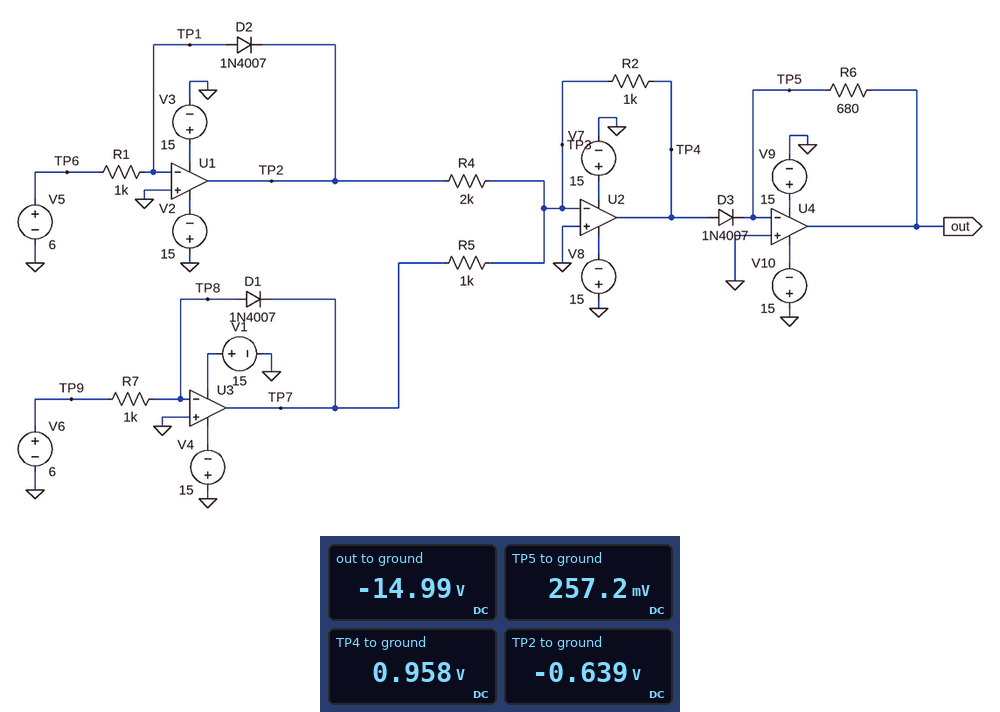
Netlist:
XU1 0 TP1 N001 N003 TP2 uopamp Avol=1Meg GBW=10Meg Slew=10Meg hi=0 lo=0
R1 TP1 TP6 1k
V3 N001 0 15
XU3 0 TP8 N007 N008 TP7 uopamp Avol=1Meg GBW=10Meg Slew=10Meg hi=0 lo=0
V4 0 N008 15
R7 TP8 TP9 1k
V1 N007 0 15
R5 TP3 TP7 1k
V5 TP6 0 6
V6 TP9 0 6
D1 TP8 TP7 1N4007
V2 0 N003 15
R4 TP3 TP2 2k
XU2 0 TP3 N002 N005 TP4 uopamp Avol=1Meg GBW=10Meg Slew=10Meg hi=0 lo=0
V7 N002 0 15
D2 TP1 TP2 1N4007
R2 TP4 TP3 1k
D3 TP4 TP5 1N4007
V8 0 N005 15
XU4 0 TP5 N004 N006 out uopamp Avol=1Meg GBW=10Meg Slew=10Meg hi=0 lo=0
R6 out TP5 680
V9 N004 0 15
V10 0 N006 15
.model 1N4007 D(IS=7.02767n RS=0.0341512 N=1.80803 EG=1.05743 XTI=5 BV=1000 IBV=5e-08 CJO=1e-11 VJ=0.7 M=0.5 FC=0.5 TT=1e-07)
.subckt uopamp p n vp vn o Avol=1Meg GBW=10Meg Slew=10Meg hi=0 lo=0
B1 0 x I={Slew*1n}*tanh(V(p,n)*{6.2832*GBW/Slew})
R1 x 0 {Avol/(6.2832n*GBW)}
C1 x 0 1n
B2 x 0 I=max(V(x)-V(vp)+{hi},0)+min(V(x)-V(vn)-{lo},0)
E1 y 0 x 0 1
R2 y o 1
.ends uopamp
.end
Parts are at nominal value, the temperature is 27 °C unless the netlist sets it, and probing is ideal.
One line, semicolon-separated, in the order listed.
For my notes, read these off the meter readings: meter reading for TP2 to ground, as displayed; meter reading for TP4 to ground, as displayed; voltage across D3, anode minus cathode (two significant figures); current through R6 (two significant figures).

-0.639 V; 0.958 V; 700 mV; 22 mA
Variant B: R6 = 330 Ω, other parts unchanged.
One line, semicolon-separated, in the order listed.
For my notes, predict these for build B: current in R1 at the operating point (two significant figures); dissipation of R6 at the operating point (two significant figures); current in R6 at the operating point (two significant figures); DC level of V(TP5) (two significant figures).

6.0 mA; 700 mW; 46 mA; 220 mV
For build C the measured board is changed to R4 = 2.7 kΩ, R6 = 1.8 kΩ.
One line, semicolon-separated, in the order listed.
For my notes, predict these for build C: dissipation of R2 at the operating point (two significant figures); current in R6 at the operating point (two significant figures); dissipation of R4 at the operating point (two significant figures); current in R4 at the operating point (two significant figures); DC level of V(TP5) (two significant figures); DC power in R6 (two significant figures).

770 µW; 8.5 mA; 150 µW; 240 µA; 220 mV; 130 mW
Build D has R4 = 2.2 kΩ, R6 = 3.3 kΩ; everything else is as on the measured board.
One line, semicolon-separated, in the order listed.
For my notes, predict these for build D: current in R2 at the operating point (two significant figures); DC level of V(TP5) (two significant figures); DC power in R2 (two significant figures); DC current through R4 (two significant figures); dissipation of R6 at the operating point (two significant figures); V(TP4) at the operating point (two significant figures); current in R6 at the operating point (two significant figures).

930 µA; 300 mV; 860 µW; 290 µA; 71 mW; 930 mV; 4.6 mA
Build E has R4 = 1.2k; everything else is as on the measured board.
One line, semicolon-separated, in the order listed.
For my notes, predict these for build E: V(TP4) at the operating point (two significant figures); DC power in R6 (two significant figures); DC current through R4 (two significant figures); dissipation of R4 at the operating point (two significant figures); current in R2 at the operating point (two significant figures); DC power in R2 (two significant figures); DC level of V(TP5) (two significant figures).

1.2 V; 350 mW; 530 µA; 340 µW; 1.2 mA; 1.4 mW; 470 mV
